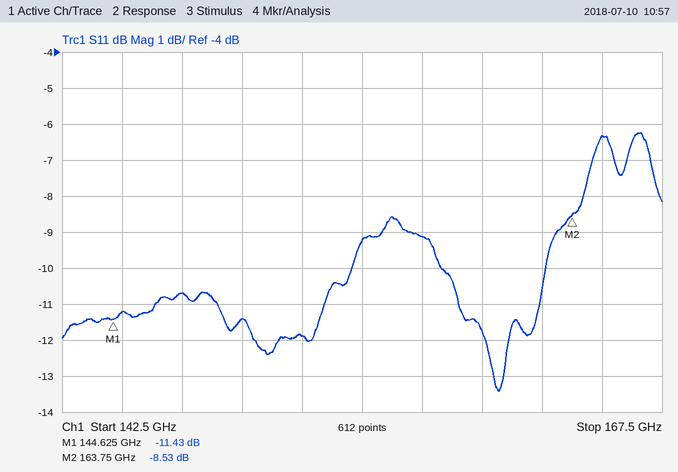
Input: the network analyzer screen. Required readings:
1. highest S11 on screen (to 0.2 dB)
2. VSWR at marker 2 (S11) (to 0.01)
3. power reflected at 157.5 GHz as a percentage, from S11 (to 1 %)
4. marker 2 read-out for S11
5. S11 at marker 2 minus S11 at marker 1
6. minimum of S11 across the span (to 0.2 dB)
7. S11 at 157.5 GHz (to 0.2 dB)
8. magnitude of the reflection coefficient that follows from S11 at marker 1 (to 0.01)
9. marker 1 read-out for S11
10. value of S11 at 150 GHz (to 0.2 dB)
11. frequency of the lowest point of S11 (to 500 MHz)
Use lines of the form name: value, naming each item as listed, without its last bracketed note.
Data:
highest S11 on screen: -6.2 dB
VSWR at marker 2 (S11): 2.20
power reflected at 157.5 GHz as a percentage, from S11: 12 %
marker 2 read-out for S11: -8.53 dB
S11 at marker 2 minus S11 at marker 1: 2.90 dB
minimum of S11 across the span: -13.4 dB
S11 at 157.5 GHz: -9.2 dB
magnitude of the reflection coefficient that follows from S11 at marker 1: 0.27
marker 1 read-out for S11: -11.43 dB
value of S11 at 150 GHz: -11.4 dB
frequency of the lowest point of S11: 160.5 GHz
